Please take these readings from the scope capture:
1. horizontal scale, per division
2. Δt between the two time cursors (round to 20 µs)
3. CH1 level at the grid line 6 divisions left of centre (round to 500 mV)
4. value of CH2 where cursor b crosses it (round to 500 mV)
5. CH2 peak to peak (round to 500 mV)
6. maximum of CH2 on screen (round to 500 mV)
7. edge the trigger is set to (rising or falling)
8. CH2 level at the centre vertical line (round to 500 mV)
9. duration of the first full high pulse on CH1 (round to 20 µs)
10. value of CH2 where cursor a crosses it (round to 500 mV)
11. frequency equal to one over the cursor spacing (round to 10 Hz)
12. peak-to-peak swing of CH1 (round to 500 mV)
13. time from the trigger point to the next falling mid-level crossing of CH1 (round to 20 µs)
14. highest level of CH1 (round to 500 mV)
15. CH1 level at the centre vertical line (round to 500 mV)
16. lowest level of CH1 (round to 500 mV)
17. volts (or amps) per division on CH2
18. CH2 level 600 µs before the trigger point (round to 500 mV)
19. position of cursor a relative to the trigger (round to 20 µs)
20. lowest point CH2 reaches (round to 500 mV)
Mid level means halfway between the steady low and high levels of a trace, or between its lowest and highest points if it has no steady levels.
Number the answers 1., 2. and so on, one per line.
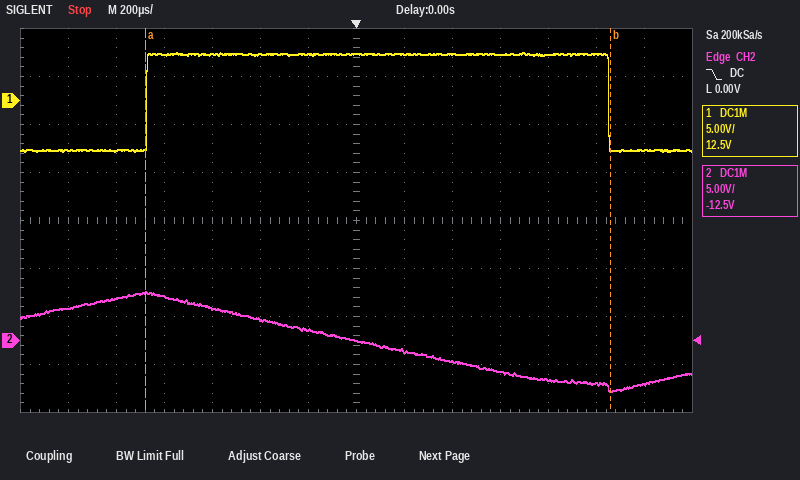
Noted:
1. 200 µs
2. 1.94 ms
3. -5.0 V
4. -5.0 V
5. 10.5 V
6. 5.0 V
7. falling
8. 0.0 V
9. 1.92 ms
10. 5.0 V
11. 520 Hz
12. 10.5 V
13. 1.06 ms
14. 5.0 V
15. 5.0 V
16. -5.5 V
17. 5 V
18. 3.5 V
19. -880 µs
20. -5.5 V
